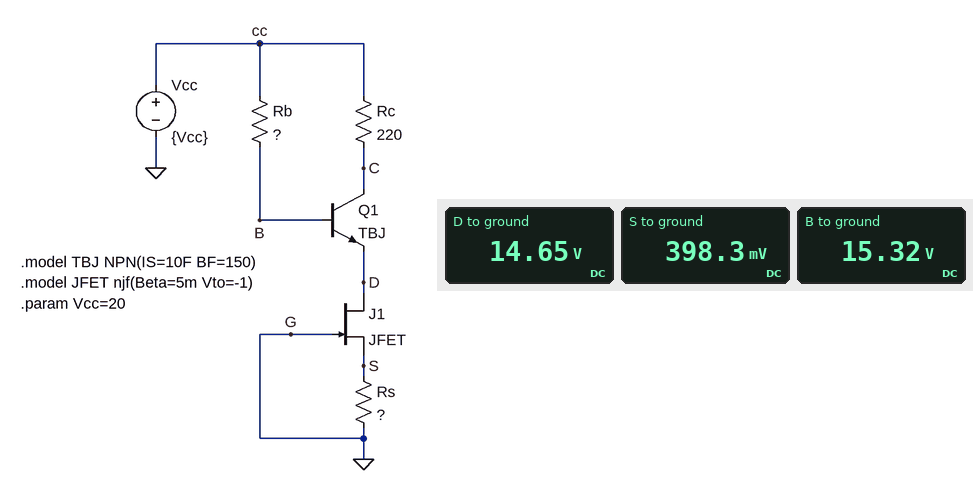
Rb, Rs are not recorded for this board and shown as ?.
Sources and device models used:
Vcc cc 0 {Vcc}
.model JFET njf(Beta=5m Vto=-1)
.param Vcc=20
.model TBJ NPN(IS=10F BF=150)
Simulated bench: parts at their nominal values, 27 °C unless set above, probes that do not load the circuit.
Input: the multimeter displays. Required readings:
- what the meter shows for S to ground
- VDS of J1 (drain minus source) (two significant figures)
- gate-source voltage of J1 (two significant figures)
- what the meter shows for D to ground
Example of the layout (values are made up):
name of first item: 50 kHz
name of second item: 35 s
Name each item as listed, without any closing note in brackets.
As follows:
what the meter shows for S to ground: 398.3 mV
VDS of J1 (drain minus source): 14 V
gate-source voltage of J1: -400 mV
what the meter shows for D to ground: 14.65 V
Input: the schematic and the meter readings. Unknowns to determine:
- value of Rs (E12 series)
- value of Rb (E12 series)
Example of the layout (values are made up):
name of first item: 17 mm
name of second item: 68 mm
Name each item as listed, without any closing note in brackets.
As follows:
value of Rs: 220 Ω
value of Rb: 390 kΩ
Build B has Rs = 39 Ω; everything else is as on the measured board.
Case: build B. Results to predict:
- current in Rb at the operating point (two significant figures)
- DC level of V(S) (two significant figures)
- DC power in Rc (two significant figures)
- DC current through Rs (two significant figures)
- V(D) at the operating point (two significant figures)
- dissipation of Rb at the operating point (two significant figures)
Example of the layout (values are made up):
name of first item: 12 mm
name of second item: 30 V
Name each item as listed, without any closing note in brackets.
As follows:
current in Rb at the operating point: 24 µA
DC level of V(S): 140 mV
DC power in Rc: 2.9 mW
DC current through Rs: 3.7 mA
V(D) at the operating point: 9.8 V
dissipation of Rb at the operating point: 230 µW
